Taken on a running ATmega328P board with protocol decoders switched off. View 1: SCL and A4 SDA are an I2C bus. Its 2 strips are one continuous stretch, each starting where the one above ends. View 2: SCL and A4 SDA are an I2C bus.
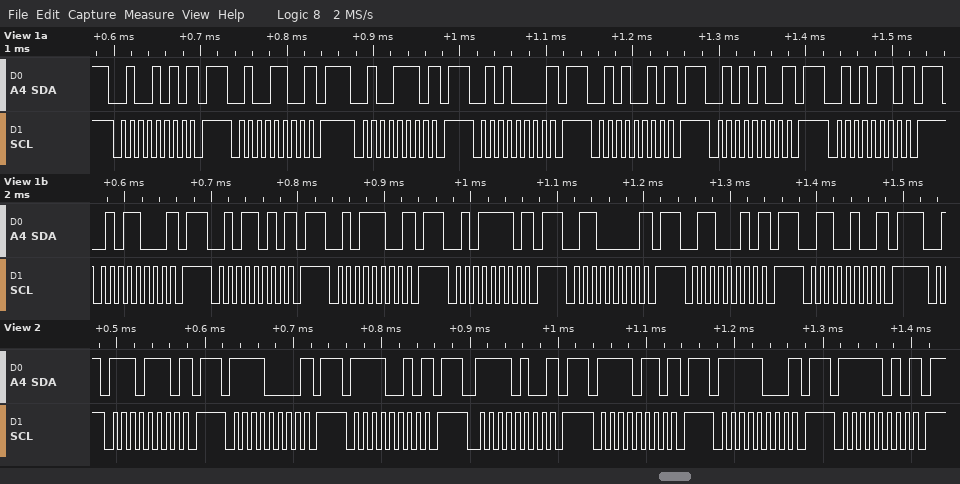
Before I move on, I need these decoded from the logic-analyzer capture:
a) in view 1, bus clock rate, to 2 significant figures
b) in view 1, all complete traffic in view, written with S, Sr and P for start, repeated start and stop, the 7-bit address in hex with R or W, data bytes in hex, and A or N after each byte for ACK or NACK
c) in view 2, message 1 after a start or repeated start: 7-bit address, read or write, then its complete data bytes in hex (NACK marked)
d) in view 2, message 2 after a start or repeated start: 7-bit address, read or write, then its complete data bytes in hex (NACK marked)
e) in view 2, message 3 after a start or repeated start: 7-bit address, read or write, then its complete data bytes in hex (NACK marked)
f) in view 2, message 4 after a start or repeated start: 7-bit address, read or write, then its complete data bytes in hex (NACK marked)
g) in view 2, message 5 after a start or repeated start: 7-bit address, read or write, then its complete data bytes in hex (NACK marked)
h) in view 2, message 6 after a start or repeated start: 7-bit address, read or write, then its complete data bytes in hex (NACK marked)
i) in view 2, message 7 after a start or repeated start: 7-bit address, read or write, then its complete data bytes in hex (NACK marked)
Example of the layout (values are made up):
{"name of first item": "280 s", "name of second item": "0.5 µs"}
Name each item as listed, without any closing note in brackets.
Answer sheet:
{"in view 1, bus clock rate, to 2 significant figures": "100 kHz", "in view 1, all complete traffic in view, written with S, Sr and P for start, repeated start and stop, the 7-bit address in hex with R or W, data bytes in hex, and A or N after each byte for ACK or NACK": "S 25W N P S 26W N P S 27W N P S 28W N P S 29W N P S 2AW N P S 2BW N P S 2CW N P S 2DW N P S 2EW N P S 2FW N P S 30W N P S 31W N P S 32W N P", "in view 2, message 1 after a start or repeated start: 7-bit address, read or write, then its complete data bytes in hex": "0x77 write NACK", "in view 2, message 2 after a start or repeated start: 7-bit address, read or write, then its complete data bytes in hex": "0x78 write NACK", "in view 2, message 3 after a start or repeated start: 7-bit address, read or write, then its complete data bytes in hex": "0x79 write NACK", "in view 2, message 4 after a start or repeated start: 7-bit address, read or write, then its complete data bytes in hex": "0x7A write NACK", "in view 2, message 5 after a start or repeated start: 7-bit address, read or write, then its complete data bytes in hex": "0x7B write NACK", "in view 2, message 6 after a start or repeated start: 7-bit address, read or write, then its complete data bytes in hex": "0x7C write NACK", "in view 2, message 7 after a start or repeated start: 7-bit address, read or write, then its complete data bytes in hex": "0x7D write NACK"}
